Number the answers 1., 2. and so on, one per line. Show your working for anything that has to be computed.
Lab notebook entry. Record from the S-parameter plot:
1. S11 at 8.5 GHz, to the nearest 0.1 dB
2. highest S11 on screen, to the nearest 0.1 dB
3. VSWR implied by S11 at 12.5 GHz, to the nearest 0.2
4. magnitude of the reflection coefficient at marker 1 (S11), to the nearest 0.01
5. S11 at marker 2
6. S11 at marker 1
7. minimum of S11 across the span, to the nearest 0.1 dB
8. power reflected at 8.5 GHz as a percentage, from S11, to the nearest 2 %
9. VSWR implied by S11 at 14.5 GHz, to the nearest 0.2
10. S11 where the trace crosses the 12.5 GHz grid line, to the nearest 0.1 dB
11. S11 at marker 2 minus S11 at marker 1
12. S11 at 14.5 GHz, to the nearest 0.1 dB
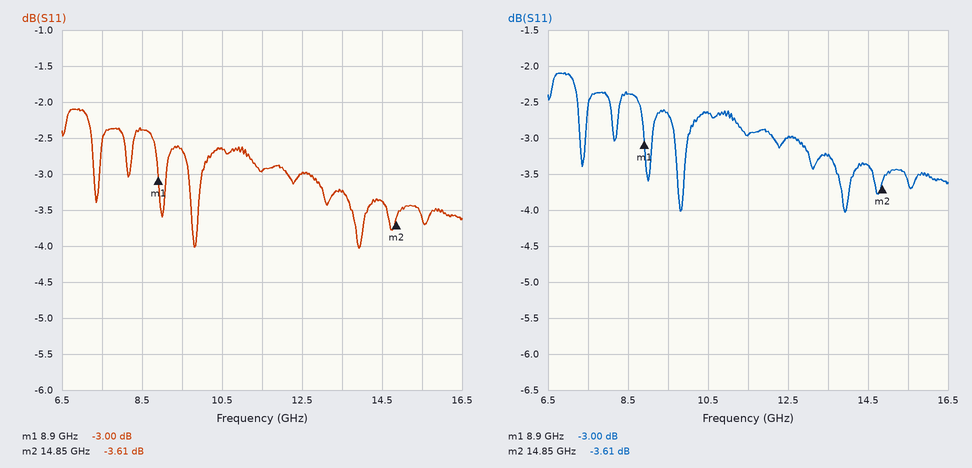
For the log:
1. -2.4 dB
2. -2.1 dB
3. |Γ| = 10^(-3/20) = 0.7079; VSWR = (1 + 0.7079)/(1 − 0.7079) ≈ 5.8
4. 10^(-3/20) ≈ 0.71
5. -3.61 dB
6. -3.00 dB
7. -4.0 dB
8. 10^(-2.4/10) ≈ 58 %
9. |Γ| = 10^(-3.4/20) = 0.6761; VSWR = (1 + 0.6761)/(1 − 0.6761) ≈ 5.2
10. -3.0 dB
11. -3.61 − (-3) = -0.61 dB
12. -3.4 dB
